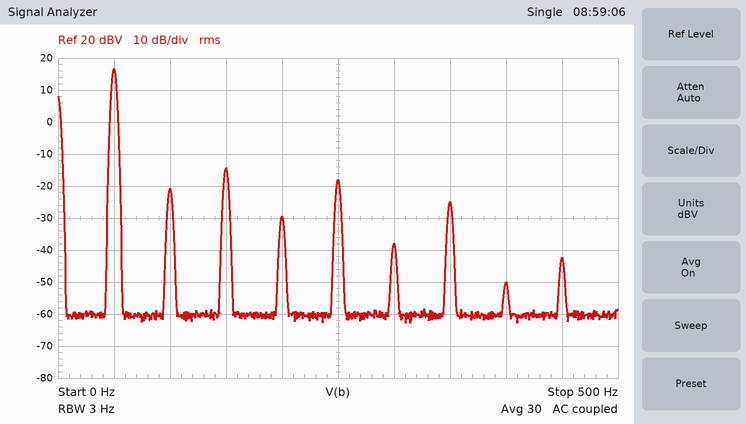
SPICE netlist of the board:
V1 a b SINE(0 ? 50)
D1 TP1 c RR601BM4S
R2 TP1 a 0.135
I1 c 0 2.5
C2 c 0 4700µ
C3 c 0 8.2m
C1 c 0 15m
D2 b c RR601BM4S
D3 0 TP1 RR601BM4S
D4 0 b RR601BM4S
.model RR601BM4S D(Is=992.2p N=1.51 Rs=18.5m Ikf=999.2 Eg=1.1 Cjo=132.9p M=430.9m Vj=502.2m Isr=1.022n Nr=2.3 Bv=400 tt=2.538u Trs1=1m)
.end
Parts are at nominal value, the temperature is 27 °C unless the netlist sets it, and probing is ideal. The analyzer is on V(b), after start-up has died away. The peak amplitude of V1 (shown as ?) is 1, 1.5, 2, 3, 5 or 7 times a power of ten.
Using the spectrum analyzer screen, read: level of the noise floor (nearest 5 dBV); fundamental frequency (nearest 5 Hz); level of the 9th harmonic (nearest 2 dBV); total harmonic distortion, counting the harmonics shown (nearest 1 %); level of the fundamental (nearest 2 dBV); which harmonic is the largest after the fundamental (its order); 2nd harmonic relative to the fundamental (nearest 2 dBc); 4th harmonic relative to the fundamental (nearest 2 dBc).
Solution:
-60 dBV
50 Hz
-42 dBV
4 %
16 dBV
3
-38 dBc
-46 dBc
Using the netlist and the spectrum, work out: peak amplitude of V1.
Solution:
20 V
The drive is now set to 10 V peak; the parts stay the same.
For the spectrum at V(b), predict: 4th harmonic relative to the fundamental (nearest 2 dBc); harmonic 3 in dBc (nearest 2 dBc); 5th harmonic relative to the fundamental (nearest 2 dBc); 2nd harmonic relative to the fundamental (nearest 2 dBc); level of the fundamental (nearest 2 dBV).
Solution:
-42 dBc
-26 dBc
-32 dBc
-32 dBc
10 dBV
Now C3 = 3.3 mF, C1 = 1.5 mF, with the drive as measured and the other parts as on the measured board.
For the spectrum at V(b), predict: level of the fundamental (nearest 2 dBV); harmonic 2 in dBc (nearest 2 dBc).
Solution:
16 dBV
-28 dBc
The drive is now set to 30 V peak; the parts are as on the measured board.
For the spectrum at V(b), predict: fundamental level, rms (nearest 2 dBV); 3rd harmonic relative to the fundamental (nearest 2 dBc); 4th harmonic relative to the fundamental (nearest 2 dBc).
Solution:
20 dBV
-34 dBc
-48 dBc
